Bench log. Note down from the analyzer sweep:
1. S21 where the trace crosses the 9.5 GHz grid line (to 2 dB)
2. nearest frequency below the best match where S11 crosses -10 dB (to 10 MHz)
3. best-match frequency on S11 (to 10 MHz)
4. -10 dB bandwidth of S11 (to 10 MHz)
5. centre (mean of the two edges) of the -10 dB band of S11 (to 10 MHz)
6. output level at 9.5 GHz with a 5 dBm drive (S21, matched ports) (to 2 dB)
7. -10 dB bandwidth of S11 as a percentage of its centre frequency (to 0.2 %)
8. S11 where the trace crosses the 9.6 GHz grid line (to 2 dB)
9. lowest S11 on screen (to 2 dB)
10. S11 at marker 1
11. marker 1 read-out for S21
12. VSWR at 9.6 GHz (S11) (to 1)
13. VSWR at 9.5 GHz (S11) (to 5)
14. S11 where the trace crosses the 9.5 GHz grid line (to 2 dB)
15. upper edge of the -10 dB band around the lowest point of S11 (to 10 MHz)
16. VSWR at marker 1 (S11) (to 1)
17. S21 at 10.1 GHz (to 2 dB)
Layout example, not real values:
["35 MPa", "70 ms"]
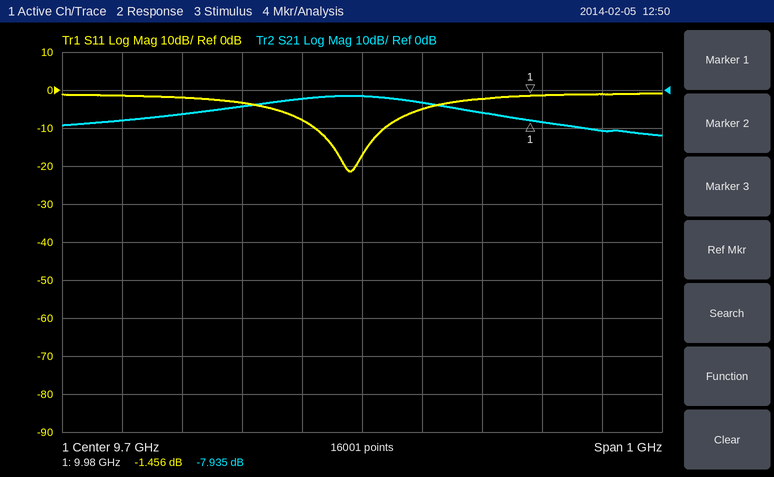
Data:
["-4 dB", "9.62 GHz", "9.68 GHz", "120 MHz", "9.68 GHz", "0 dBm", "1.2 %", "-8 dB", "-22 dB", "-1.456 dB", "-7.935 dB", "2", "5", "-4 dB", "9.74 GHz", "12", "-10 dB"]
